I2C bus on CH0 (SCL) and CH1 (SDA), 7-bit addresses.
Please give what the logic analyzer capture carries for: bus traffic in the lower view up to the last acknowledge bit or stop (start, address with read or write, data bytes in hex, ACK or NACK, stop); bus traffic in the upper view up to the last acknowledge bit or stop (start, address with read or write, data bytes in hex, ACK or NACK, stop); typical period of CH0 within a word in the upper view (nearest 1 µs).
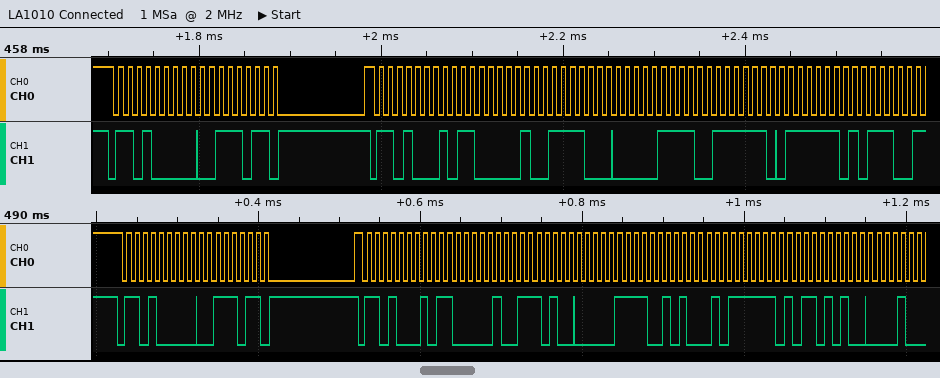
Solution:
start, address 68 write ACK, 3B ACK, repeated start, address 68 read ACK, C1 ACK, 74 ACK, 0F ACK, 51 ACK, FD ACK, D4 ACK
start, address 68 write ACK, 3B ACK, repeated start, address 68 read ACK, C1 ACK, 78 ACK, 0F ACK, 7E ACK, FD ACK
10 µs
